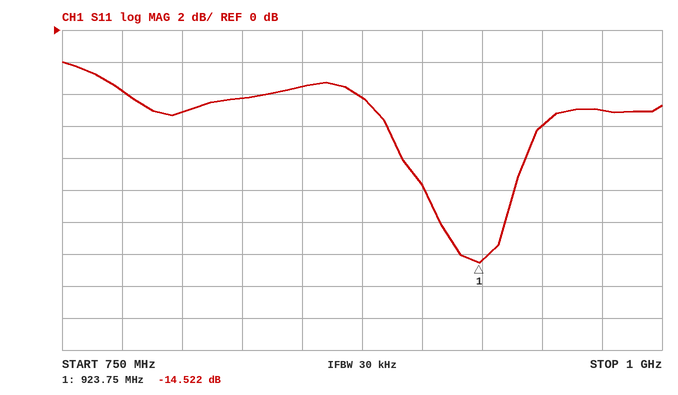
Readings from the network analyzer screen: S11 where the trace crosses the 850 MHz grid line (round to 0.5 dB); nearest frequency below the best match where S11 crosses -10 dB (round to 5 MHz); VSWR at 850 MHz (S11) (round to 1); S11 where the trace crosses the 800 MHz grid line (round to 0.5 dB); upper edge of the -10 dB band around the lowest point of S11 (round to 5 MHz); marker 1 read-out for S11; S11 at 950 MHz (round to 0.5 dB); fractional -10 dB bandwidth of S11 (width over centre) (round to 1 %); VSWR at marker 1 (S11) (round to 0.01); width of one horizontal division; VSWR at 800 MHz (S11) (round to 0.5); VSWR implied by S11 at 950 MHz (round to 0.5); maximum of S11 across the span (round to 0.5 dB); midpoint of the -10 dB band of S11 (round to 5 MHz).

-3.5 dB
900 MHz
5
-5.0 dB
940 MHz
-14.522 dB
-6.0 dB
4 %
1.46
25 MHz
3.5
3.0
-2.0 dB
920 MHz
